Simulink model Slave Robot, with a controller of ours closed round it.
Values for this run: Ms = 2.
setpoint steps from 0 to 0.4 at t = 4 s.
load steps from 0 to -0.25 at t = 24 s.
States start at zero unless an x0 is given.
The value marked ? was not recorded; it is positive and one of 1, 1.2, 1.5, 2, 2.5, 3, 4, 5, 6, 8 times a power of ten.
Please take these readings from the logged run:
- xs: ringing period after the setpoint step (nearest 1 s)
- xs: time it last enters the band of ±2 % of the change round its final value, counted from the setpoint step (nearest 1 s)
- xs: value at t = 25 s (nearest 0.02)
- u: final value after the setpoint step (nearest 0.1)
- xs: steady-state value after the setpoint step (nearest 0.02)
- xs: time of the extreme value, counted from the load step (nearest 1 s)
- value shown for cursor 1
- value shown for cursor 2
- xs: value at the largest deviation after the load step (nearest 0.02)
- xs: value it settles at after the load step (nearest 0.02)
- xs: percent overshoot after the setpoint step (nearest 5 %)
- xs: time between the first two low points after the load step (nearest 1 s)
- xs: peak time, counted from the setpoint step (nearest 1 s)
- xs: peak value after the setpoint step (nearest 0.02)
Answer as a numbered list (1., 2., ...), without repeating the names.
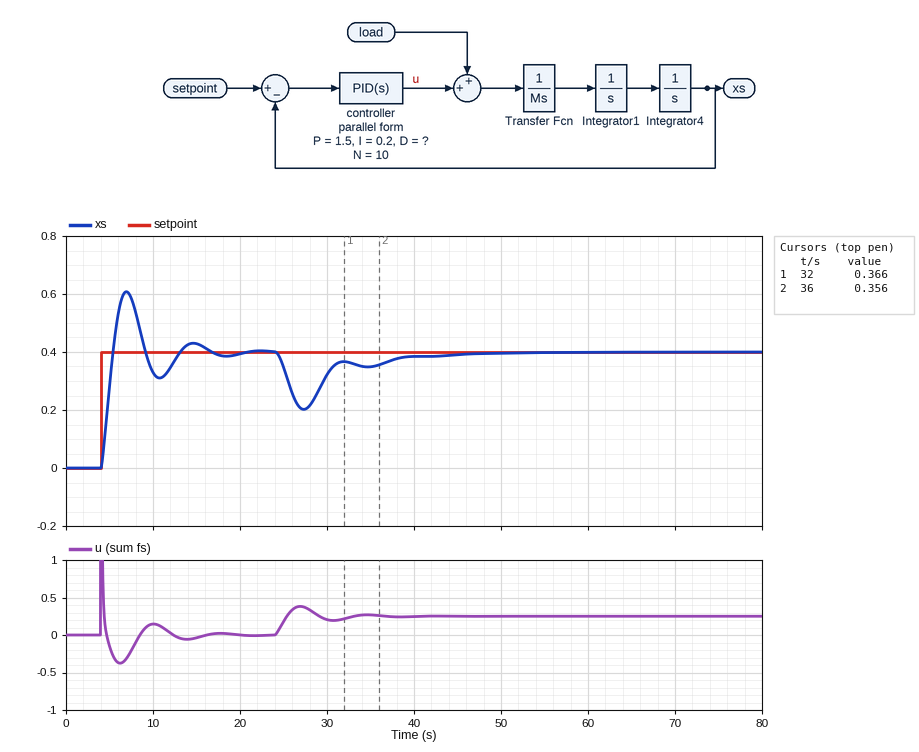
1. 8 s
2. 16 s
3. 0.34
4. 0.0
5. 0.40
6. 3 s
7. 0.366
8. 0.356
9. 0.20
10. 0.40
11. 50 %
12. 7 s
13. 3 s
14. 0.60
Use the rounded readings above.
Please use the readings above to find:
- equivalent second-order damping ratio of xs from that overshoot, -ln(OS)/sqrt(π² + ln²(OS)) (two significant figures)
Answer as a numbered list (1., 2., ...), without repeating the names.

1. 0.22
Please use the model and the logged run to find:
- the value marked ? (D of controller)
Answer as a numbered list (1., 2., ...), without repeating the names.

1. 1.2
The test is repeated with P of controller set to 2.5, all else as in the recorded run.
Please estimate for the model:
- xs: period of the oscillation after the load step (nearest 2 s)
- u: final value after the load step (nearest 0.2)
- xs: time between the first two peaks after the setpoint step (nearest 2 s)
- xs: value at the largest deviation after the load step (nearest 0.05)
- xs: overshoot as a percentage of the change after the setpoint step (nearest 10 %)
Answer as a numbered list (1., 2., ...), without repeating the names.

1. 6 s
2. 0.2
3. 6 s
4. 0.25
5. 60 %
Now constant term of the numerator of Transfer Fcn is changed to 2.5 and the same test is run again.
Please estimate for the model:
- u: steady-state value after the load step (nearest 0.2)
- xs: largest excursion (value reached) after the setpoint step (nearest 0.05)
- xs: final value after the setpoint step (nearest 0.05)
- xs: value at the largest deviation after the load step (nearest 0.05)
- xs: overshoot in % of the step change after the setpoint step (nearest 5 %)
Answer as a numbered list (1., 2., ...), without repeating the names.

1. 0.2
2. 0.55
3. 0.40
4. 0.25
5. 35 %
